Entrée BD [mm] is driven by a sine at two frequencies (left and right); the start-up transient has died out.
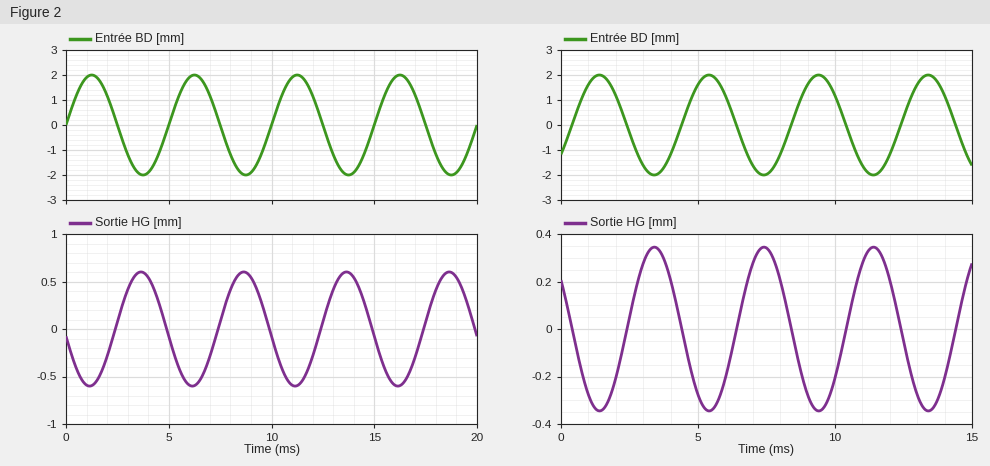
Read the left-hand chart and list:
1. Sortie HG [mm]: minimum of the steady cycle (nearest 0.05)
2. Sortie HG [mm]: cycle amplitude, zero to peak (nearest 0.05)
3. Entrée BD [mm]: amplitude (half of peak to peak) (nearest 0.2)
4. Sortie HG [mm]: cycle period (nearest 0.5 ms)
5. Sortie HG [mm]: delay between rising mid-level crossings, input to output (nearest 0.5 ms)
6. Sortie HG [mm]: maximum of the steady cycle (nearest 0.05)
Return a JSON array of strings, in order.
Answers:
["-0.60", "0.60", "2.0", "5.0 ms", "2.5 ms", "0.60"]
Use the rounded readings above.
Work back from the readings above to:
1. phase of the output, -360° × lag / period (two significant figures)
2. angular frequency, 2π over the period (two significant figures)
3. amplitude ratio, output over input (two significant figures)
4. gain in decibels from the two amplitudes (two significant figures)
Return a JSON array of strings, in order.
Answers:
["-180°", "1.3 rad/ms", "0.30", "-10 dB"]
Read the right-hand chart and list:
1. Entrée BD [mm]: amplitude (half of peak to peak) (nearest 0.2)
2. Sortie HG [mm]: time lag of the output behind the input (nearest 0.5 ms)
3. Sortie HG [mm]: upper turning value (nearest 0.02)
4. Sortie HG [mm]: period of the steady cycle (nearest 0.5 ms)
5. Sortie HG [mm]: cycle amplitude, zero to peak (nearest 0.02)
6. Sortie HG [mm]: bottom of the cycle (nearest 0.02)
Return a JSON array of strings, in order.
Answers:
["2.0", "2.0 ms", "0.34", "4.0 ms", "0.34", "-0.34"]
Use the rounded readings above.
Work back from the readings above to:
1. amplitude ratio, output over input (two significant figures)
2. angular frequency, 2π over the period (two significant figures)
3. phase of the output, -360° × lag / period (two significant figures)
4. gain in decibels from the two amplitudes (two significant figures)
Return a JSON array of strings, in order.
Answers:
["0.17", "1.6 rad/ms", "-180°", "-15 dB"]
